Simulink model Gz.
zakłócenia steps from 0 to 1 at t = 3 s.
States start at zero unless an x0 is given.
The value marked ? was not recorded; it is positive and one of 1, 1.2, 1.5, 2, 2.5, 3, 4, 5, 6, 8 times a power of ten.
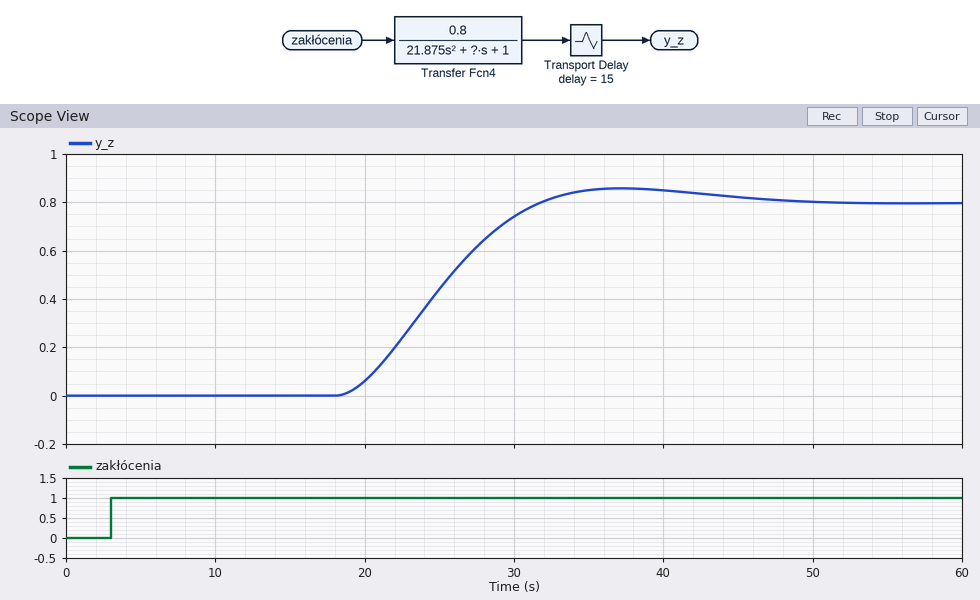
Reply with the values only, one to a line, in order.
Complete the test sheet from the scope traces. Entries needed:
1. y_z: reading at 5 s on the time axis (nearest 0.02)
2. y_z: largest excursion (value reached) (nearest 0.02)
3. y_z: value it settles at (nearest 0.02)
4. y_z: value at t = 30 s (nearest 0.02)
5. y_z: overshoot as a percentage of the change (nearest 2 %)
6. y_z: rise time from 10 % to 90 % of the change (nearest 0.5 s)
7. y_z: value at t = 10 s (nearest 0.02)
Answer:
0.00
0.86
0.80
0.74
8 %
9.0 s
0.00
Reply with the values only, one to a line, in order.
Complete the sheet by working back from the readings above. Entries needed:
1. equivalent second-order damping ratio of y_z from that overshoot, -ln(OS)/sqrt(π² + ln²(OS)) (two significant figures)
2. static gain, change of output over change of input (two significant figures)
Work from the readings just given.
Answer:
0.63
0.80
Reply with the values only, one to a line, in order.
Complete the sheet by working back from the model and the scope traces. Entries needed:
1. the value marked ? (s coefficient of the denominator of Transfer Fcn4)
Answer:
6
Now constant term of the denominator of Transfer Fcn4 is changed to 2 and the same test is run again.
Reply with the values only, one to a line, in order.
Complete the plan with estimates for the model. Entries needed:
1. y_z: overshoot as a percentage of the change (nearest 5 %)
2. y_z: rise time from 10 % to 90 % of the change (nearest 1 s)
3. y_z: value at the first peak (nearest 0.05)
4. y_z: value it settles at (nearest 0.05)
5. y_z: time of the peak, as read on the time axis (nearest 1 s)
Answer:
20 %
5 s
0.50
0.40
30 s
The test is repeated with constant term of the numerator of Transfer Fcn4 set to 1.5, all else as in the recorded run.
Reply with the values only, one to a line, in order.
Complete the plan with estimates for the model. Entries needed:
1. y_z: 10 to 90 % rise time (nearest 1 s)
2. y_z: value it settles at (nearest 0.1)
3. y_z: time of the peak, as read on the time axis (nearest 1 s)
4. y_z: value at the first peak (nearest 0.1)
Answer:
9 s
1.5
37 s
1.6
